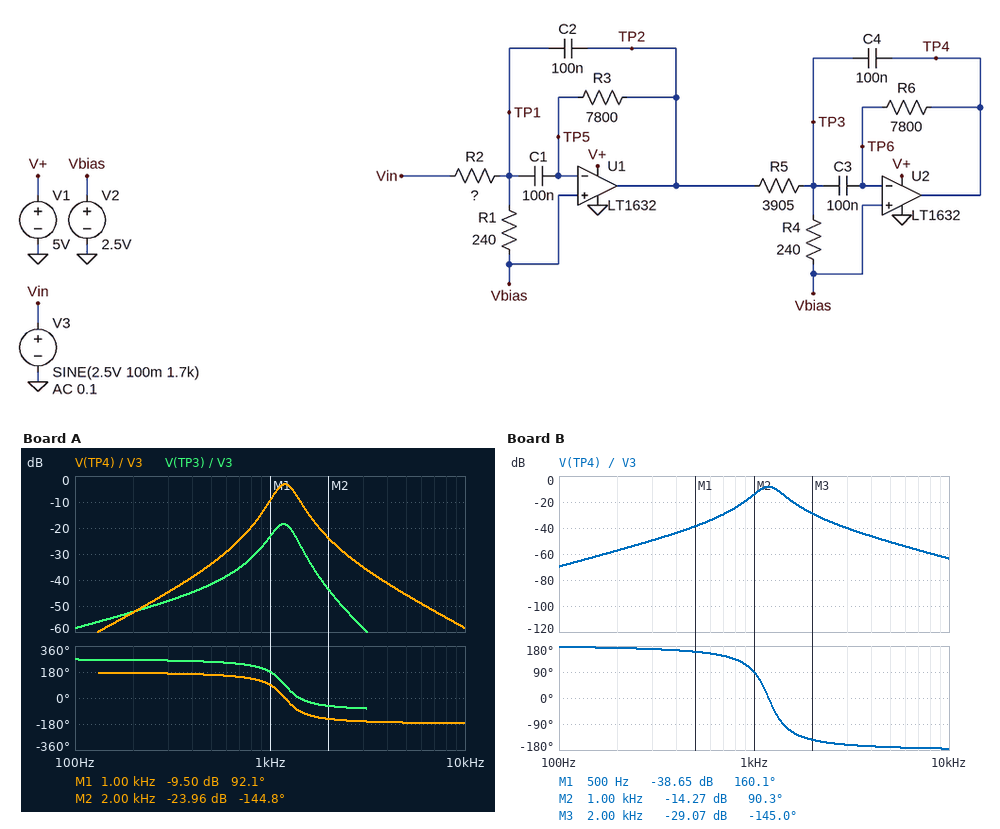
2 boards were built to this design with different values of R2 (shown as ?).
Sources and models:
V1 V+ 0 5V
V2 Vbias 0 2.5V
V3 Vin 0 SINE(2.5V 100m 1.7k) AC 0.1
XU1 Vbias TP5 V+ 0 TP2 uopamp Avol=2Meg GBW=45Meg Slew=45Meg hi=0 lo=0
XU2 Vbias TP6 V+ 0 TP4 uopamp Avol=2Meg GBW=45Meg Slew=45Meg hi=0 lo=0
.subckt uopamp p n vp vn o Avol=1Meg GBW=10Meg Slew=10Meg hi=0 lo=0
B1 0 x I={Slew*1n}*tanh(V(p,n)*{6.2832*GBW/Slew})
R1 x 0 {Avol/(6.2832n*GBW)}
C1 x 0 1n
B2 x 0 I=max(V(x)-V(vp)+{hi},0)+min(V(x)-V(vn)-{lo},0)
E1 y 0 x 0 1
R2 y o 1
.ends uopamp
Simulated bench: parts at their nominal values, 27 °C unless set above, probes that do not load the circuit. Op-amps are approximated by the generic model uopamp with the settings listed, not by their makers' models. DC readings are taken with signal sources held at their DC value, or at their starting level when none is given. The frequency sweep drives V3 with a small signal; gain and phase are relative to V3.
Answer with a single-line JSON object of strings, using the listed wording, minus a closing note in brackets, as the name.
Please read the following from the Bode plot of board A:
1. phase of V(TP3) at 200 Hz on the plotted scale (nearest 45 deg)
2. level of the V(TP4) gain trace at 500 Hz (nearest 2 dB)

{"phase of V(TP3) at 200 Hz on the plotted scale": "270 deg", "level of the V(TP4) gain trace at 500 Hz": "-34 dB"}
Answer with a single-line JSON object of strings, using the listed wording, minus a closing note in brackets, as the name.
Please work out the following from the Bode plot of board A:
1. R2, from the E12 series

{"R2, from the E12 series": "5.6 kΩ"}
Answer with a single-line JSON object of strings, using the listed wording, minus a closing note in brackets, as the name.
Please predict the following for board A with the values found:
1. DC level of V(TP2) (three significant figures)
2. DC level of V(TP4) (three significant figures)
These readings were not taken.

{"DC level of V(TP2)": "2.50 V", "DC level of V(TP4)": "2.50 V"}
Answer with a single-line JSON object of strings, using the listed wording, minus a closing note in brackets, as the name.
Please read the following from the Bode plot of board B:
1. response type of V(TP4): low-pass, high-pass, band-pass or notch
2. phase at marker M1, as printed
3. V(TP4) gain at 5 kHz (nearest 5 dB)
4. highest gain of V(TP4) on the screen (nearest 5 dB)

{"response type of V(TP4): low-pass, high-pass, band-pass or notch": "band-pass", "phase at marker M1, as printed": "160.1 deg", "V(TP4) gain at 5 kHz": "-50 dB", "highest gain of V(TP4) on the screen": "-10 dB"}
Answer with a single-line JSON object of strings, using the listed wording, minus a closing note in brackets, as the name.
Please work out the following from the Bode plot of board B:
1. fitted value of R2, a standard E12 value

{"fitted value of R2, a standard E12 value": "10 kΩ"}
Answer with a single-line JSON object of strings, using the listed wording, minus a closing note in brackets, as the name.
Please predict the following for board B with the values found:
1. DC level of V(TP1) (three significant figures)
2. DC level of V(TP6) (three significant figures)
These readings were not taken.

{"DC level of V(TP1)": "2.50 V", "DC level of V(TP6)": "2.50 V"}
